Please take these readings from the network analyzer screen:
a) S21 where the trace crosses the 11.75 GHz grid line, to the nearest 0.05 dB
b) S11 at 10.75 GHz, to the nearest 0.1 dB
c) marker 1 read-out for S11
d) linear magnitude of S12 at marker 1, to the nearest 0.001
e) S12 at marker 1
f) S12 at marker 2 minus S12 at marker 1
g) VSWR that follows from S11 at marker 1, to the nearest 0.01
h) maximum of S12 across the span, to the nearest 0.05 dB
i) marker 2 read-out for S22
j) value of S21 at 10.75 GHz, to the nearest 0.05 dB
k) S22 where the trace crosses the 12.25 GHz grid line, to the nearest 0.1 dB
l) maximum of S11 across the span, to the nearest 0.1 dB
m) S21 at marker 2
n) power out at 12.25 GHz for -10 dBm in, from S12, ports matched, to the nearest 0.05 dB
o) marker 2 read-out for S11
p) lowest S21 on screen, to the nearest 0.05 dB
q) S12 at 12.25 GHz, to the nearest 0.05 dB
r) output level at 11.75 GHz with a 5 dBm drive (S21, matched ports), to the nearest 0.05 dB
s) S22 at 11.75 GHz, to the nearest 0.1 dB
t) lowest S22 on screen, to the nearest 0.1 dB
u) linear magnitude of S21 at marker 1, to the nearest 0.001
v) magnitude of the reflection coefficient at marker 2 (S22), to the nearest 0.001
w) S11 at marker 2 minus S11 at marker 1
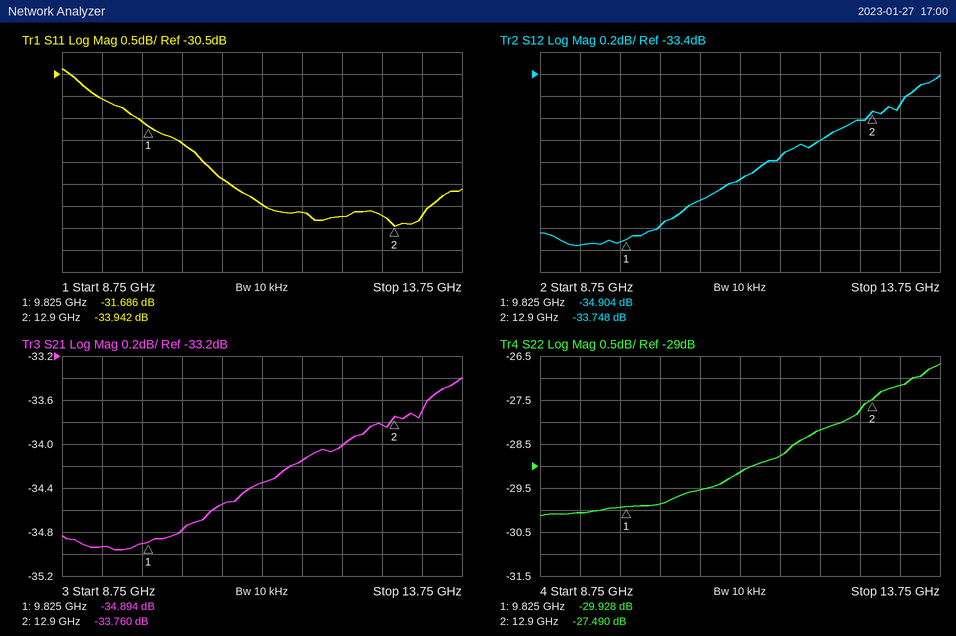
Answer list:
-34.15 dB
-32.9 dB
-31.686 dB
0.018
-34.904 dB
1.156 dB
1.05
-33.40 dB
-27.490 dB
-34.55 dB
-28.2 dB
-30.4 dB
-33.760 dB
-44.00 dBm
-33.942 dB
-34.95 dB
-34.00 dB
-29.15 dBm
-28.8 dB
-30.1 dB
0.018
0.042
-2.256 dB
